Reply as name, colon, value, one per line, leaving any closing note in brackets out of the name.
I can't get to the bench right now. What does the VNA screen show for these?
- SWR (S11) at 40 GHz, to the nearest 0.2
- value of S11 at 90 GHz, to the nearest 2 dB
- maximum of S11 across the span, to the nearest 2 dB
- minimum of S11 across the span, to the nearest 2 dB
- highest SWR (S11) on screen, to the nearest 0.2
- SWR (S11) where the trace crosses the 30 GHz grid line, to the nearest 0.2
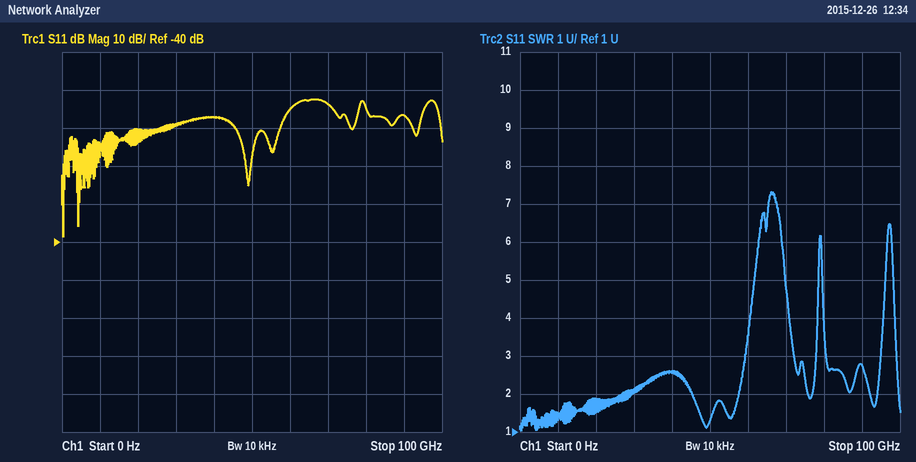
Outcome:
SWR (S11) at 40 GHz, to the nearest 0.2: 2.6
value of S11 at 90 GHz, to the nearest 2 dB: -6 dB
maximum of S11 across the span, to the nearest 2 dB: -2 dB
minimum of S11 across the span, to the nearest 2 dB: -38 dB
highest SWR (S11) on screen, to the nearest 0.2: 7.4
SWR (S11) where the trace crosses the 30 GHz grid line, to the nearest 0.2: 2.0
